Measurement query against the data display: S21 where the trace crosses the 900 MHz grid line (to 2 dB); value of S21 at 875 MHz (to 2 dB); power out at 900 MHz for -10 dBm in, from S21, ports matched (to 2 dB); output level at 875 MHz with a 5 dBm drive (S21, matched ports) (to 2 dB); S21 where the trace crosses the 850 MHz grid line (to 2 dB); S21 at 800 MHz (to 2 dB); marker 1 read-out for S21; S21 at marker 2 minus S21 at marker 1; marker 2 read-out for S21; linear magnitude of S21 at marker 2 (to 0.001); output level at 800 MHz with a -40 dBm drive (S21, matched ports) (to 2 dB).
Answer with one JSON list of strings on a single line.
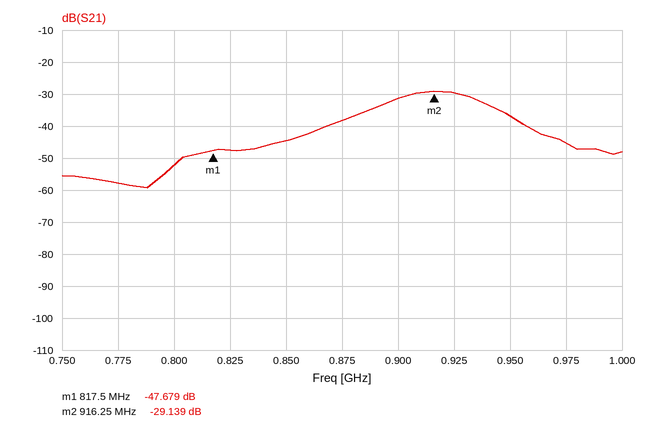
["-32 dB", "-38 dB", "-42 dBm", "-34 dBm", "-44 dB", "-52 dB", "-47.679 dB", "18.540 dB", "-29.139 dB", "0.035", "-92 dBm"]
